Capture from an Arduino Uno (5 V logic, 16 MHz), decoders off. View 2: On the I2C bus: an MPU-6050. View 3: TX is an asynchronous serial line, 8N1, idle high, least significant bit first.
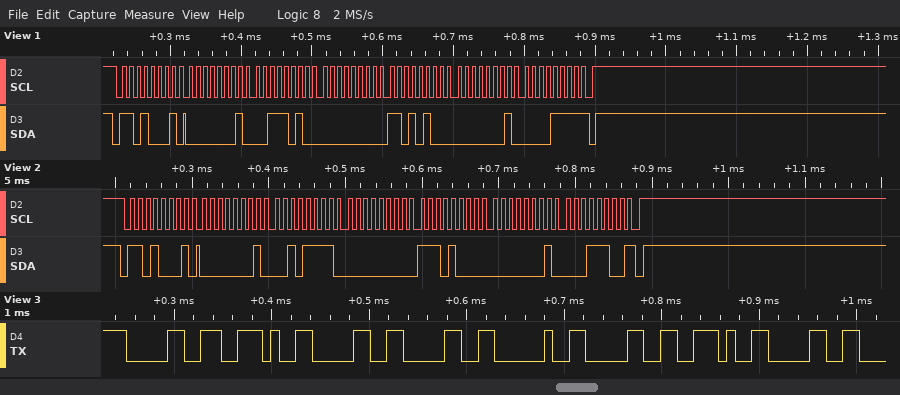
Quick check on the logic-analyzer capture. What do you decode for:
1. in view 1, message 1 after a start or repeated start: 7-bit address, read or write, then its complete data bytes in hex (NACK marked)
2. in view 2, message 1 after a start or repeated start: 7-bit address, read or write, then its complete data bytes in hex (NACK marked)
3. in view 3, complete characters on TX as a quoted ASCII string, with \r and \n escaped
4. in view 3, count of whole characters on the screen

0x68 read: 01 3A 00 D4 01 0F NACK
0x68 read: 01 2F 00 E8 01 1C NACK
"0.00 0.0"
8
